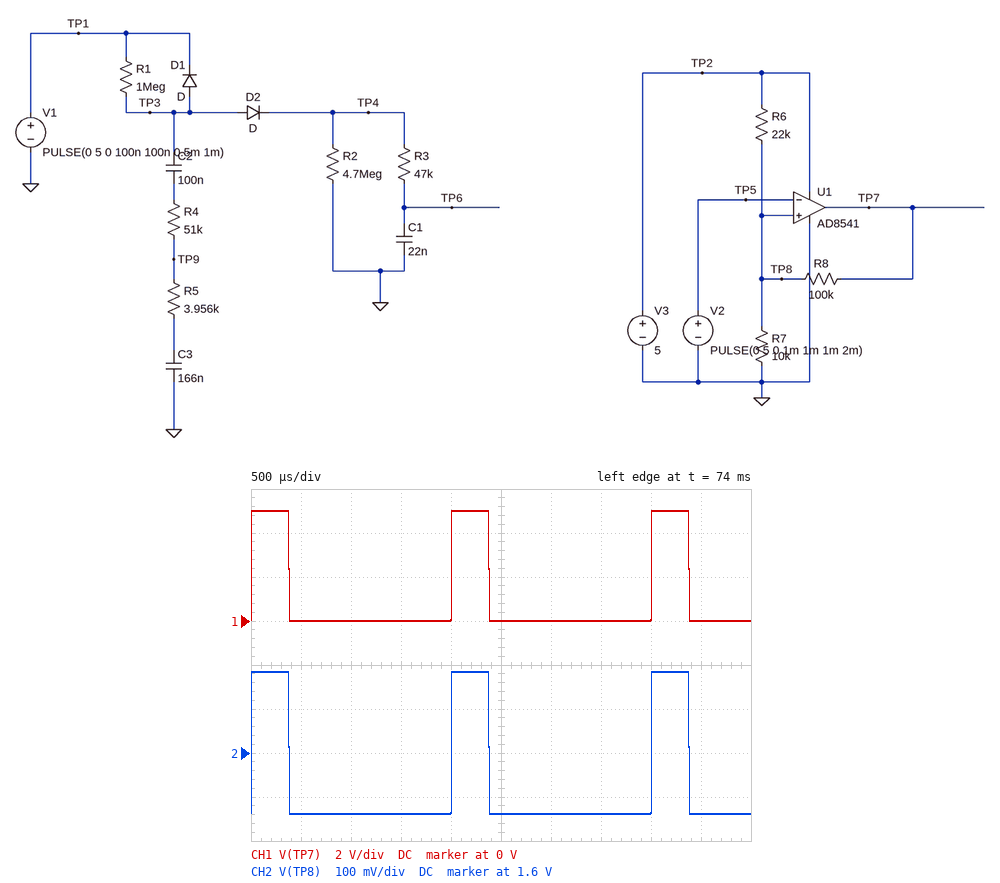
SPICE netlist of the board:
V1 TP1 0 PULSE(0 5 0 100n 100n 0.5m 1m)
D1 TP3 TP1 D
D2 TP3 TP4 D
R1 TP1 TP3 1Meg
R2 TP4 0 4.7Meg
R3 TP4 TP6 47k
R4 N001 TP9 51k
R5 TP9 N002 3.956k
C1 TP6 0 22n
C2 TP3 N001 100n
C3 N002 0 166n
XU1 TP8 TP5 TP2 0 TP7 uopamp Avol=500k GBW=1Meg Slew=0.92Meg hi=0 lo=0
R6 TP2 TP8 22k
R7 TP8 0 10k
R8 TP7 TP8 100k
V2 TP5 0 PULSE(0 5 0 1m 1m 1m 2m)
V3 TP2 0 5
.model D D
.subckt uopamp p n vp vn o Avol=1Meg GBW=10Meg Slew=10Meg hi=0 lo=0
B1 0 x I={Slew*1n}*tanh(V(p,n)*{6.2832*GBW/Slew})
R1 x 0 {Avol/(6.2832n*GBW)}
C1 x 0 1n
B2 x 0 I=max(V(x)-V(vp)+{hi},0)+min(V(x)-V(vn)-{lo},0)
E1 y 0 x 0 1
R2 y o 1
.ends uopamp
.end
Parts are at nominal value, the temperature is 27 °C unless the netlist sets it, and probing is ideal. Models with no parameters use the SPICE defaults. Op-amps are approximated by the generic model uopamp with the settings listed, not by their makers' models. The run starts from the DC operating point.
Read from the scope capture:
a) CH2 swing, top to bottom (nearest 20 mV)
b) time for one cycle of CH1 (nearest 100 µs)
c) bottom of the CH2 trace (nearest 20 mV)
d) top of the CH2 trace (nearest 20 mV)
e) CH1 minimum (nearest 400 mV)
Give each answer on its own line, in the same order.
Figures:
320 mV
2.0 ms
1.46 V
1.78 V
0 V
